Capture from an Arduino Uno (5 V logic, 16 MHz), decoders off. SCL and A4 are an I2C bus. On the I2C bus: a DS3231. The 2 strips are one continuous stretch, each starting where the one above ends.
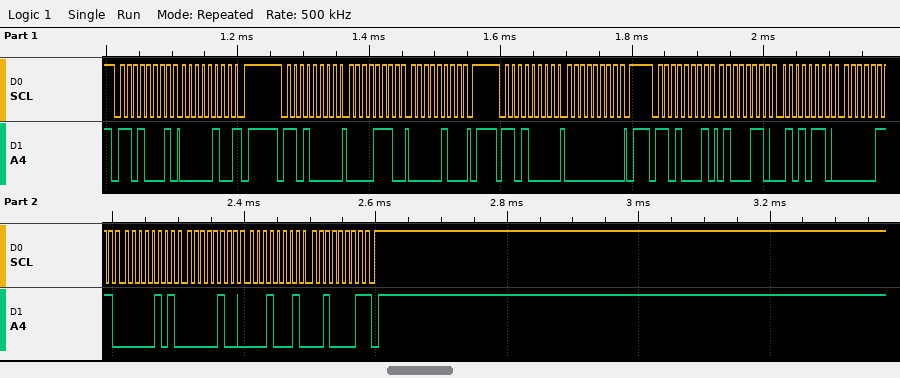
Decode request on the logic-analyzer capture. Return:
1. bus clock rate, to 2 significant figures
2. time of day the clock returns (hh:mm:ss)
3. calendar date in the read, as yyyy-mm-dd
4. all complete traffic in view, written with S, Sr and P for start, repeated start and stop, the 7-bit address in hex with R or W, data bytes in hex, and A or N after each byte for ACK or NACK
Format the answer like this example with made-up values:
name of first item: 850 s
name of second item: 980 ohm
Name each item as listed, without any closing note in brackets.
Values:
bus clock rate, to 2 significant figures: 100 kHz
time of day the clock returns: 07:56:46
calendar date in the read, as yyyy-mm-dd: 2021-11-04
all complete traffic in view, written with S, Sr and P for start, repeated start and stop, the 7-bit address in hex with R or W, data bytes in hex, and A or N after each byte for ACK or NACK: S 68R A 04 N P S 68W A 0E A 04 A P S 68W A 00 A P S 68R A 46 A 56 A 07 A 05 A 04 A 11 A 21 N P
